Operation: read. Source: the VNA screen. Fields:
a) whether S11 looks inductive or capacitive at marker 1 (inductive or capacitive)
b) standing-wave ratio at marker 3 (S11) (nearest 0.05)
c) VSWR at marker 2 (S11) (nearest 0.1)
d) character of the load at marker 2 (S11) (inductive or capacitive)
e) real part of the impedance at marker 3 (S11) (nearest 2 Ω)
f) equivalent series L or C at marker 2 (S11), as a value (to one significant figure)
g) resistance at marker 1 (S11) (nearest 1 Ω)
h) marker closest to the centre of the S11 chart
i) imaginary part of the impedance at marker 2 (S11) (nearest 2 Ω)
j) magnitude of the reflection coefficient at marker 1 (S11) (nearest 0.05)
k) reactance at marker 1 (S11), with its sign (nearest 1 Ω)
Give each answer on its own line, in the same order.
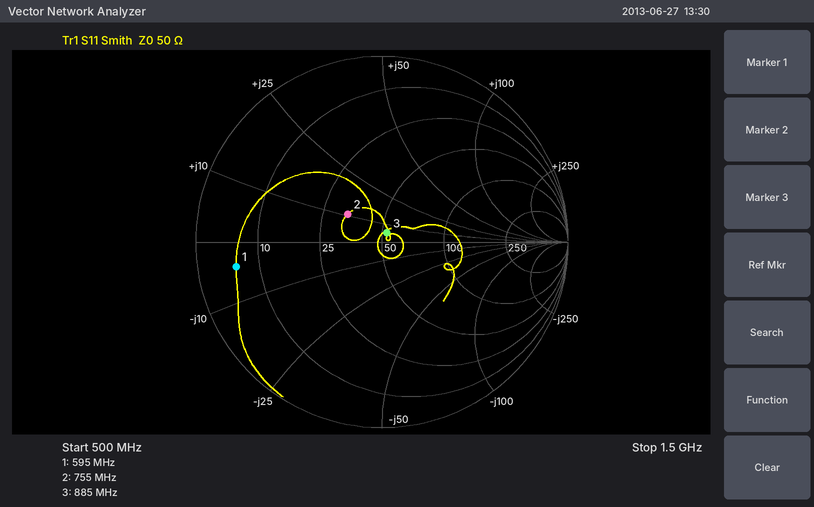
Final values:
capacitive
1.10
1.6
inductive
52 Ω
2 nH
6 Ω
marker 3
+10 Ω
0.80
-4 Ω
